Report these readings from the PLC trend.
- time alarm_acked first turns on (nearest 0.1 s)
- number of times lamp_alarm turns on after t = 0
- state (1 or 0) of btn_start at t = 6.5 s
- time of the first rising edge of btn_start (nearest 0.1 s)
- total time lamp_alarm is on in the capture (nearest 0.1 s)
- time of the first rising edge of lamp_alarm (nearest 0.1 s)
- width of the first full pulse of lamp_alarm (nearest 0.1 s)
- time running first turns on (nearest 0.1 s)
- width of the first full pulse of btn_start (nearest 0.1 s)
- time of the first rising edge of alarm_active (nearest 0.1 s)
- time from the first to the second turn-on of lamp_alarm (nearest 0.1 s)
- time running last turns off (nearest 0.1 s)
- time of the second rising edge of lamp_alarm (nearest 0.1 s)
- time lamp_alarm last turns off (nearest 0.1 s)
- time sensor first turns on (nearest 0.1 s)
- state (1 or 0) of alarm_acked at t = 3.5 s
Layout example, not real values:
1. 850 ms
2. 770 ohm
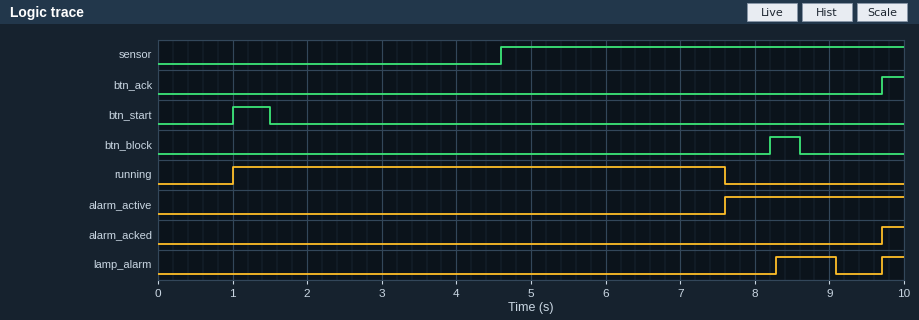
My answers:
1. 9.7 s
2. 2
3. 0
4. 1.0 s
5. 1.1 s
6. 8.3 s
7. 0.8 s
8. 1.0 s
9. 0.5 s
10. 7.6 s
11. 1.4 s
12. 7.6 s
13. 9.7 s
14. 9.1 s
15. 4.6 s
16. 0
